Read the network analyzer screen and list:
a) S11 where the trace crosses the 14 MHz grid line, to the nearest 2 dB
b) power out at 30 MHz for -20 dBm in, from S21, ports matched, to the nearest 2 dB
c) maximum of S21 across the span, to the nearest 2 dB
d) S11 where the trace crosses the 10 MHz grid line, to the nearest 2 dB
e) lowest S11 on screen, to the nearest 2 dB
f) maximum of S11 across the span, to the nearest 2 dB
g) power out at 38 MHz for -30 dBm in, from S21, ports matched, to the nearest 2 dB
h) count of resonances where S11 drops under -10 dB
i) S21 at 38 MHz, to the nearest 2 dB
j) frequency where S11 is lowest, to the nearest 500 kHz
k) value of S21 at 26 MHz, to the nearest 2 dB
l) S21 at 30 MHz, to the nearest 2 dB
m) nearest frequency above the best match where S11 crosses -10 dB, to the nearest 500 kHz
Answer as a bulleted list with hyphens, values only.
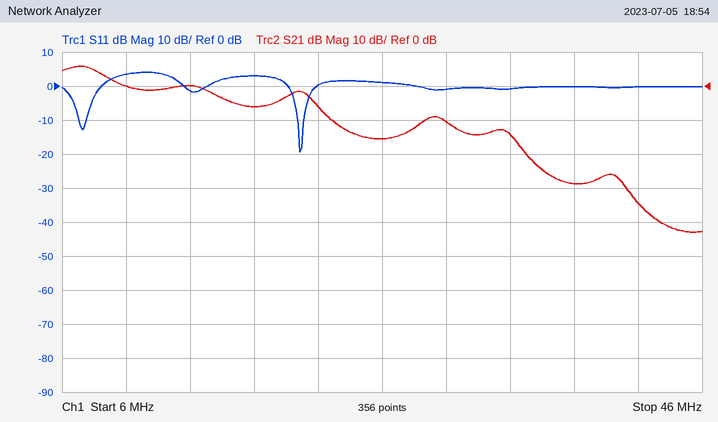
- -2 dB
- -30 dBm
- 6 dB
- 4 dB
- -20 dB
- 4 dB
- -58 dBm
- 2
- -28 dB
- 21.0 MHz
- -16 dB
- -10 dB
- 21.0 MHz
